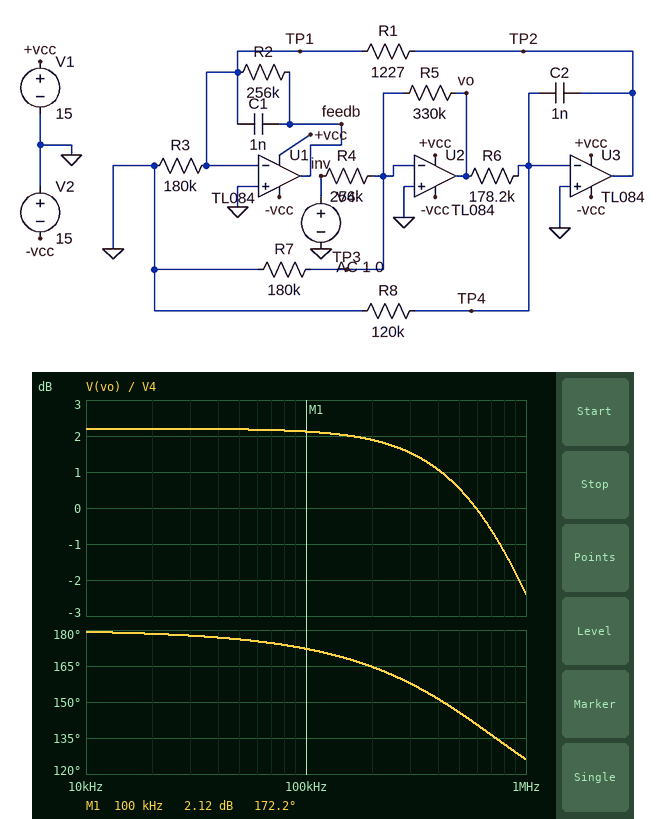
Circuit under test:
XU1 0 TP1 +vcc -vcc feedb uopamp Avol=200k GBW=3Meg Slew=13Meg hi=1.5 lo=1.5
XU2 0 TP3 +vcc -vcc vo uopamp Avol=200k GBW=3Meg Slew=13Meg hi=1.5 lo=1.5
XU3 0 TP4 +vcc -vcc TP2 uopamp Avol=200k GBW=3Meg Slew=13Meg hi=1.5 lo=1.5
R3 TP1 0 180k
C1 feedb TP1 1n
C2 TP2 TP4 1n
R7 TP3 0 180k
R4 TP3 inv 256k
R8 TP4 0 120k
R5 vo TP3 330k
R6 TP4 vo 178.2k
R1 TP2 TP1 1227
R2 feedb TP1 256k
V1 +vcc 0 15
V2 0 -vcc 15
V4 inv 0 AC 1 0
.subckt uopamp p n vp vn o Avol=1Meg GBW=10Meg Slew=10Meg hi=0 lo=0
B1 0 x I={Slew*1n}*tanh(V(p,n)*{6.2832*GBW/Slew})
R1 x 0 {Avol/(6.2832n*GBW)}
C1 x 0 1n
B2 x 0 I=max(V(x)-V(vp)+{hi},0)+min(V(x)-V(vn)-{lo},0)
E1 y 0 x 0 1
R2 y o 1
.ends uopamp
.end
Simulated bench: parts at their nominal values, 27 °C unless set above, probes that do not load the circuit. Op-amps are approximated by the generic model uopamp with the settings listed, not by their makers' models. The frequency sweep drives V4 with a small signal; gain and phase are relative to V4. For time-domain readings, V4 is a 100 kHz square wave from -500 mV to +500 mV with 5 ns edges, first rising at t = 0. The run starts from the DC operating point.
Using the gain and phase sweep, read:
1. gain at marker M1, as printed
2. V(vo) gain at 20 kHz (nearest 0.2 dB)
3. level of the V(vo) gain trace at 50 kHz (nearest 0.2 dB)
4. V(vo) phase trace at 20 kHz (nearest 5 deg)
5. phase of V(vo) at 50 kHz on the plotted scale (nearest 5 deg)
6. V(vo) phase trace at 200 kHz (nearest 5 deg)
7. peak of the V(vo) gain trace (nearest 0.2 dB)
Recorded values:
2.12 dB
2.2 dB
2.2 dB
180 deg
175 deg
165 deg
2.2 dB
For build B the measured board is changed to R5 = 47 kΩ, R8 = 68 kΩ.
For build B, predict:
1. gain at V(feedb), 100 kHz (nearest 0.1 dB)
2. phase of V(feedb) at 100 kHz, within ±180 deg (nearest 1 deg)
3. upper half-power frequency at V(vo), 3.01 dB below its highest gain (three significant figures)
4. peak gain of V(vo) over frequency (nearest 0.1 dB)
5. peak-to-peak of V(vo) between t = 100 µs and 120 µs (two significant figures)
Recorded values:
-53.8 dB
-6 deg
2.08 MHz
-14.7 dB
180 mV
